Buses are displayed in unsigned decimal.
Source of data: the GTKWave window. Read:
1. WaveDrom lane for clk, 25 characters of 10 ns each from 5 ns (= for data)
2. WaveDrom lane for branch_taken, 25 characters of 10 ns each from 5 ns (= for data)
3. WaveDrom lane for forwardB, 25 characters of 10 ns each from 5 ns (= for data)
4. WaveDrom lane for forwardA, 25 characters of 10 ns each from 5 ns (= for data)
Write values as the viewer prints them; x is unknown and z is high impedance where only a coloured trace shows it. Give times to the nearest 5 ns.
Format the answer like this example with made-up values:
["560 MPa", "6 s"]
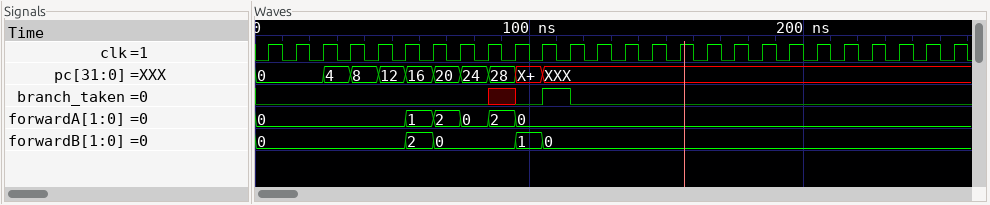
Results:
["{name: 'clk', wave: 'p........................'}", "{name: 'branch_taken', wave: '0.......x010.............'}", "{name: 'forwardB', wave: '=....==..==..............', data: '0 2 0 1 0'}", "{name: 'forwardA', wave: '=....=====...............', data: '0 1 2 0 2 0'}"]
